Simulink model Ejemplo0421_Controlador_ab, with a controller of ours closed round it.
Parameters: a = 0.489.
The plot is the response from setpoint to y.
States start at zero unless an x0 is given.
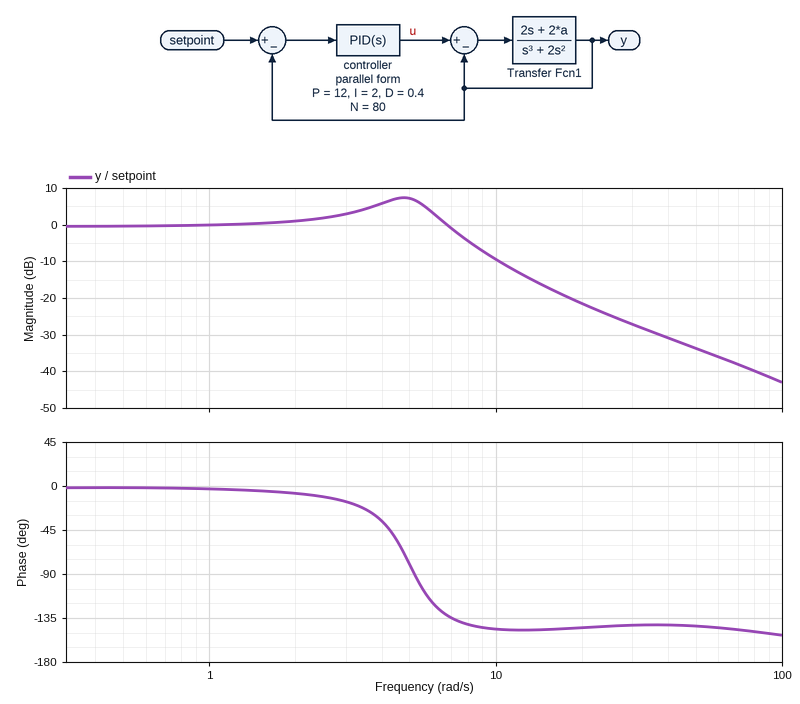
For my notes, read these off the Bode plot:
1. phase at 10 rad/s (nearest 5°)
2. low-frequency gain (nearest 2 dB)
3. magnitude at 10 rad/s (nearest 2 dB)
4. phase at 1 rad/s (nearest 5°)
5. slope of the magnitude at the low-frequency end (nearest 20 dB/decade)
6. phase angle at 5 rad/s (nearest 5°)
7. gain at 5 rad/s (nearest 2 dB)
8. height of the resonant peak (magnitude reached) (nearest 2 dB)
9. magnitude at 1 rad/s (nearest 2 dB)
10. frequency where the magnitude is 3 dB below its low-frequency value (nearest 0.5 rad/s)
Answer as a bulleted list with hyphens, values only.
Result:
- -145°
- 0 dB
- -10 dB
- -5°
- 0 dB/decade
- -80°
- 8 dB
- 8 dB
- 0 dB
- 7.5 rad/s
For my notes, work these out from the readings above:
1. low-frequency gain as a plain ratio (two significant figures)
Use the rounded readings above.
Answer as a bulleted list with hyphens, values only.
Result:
- 1.0
